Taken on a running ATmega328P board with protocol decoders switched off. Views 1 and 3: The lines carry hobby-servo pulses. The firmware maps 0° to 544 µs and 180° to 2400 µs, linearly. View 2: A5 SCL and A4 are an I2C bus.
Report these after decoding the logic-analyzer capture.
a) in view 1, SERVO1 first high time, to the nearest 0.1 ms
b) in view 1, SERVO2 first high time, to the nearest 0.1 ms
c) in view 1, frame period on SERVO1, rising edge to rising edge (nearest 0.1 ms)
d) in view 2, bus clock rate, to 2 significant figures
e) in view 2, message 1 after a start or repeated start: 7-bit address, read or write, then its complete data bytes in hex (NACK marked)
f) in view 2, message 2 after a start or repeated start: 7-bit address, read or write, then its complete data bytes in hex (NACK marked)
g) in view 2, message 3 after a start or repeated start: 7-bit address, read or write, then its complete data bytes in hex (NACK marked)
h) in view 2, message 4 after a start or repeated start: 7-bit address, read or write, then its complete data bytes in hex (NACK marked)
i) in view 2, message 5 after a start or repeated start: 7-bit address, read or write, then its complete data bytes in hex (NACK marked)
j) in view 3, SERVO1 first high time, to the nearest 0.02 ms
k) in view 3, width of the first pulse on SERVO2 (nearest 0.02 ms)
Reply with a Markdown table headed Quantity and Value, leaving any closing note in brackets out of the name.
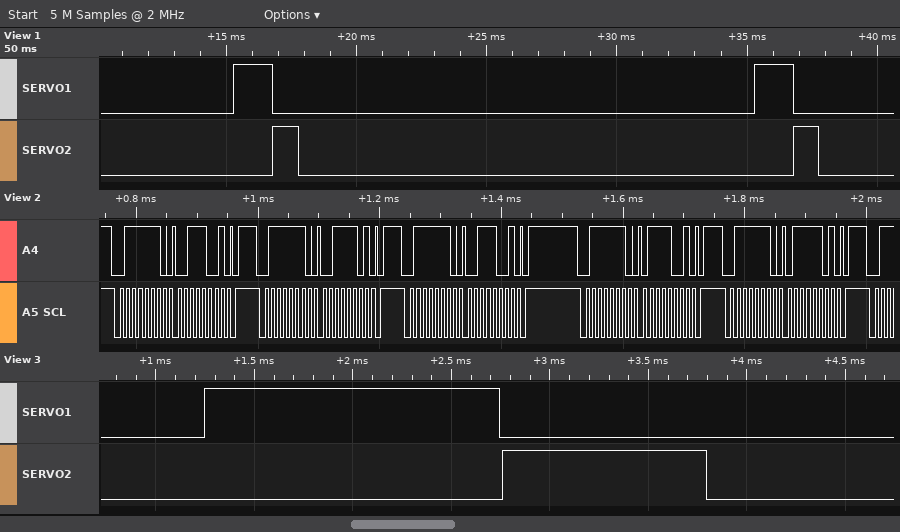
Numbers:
| Quantity | Value |
|---|---|
| in view 1, SERVO1 first high time, to the nearest 0.1 ms | 1.5 ms |
| in view 1, SERVO2 first high time, to the nearest 0.1 ms | 1.0 ms |
| in view 1, frame period on SERVO1, rising edge to rising edge | 20.0 ms |
| in view 2, bus clock rate, to 2 significant figures | 100 kHz |
| in view 2, message 1 after a start or repeated start: 7-bit address, read or write, then its complete data bytes in hex | 0x3F write: 39 |
| in view 2, message 2 after a start or repeated start: 7-bit address, read or write, then its complete data bytes in hex | 0x3F write: 3D |
| in view 2, message 3 after a start or repeated start: 7-bit address, read or write, then its complete data bytes in hex | 0x3F write: 39 |
| in view 2, message 4 after a start or repeated start: 7-bit address, read or write, then its complete data bytes in hex | 0x3F write: 79 |
| in view 2, message 5 after a start or repeated start: 7-bit address, read or write, then its complete data bytes in hex | 0x3F write: 7D |
| in view 3, SERVO1 first high time, to the nearest 0.02 ms | 1.50 ms |
| in view 3, width of the first pulse on SERVO2 | 1.04 ms |
